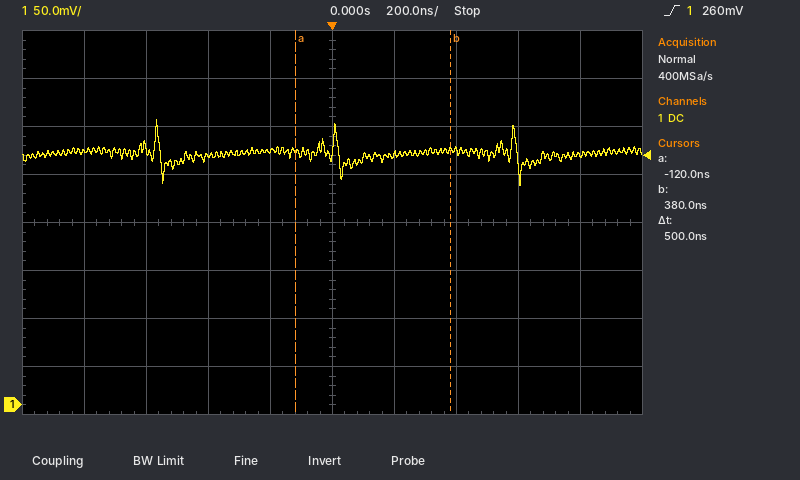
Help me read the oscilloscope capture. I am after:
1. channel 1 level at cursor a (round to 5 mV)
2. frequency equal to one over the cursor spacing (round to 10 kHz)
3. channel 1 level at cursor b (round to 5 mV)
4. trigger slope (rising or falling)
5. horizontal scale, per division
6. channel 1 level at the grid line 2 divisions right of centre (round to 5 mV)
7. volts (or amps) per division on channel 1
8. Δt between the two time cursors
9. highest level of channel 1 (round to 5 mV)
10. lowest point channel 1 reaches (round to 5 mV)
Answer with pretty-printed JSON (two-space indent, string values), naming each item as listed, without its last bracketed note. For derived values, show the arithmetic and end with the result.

{
  "channel 1 level at cursor a": "265 mV",
  "frequency equal to one over the cursor spacing": "1 / 500 ns ≈ 2.00 MHz",
  "channel 1 level at cursor b": "265 mV",
  "trigger slope": "rising",
  "horizontal scale, per division": "200 ns",
  "channel 1 level at the grid line 2 divisions right of centre": "265 mV",
  "volts (or amps) per division on channel 1": "50 mV",
  "Δt between the two time cursors": "500 ns",
  "highest level of channel 1": "295 mV",
  "lowest point channel 1 reaches": "230 mV"
}
